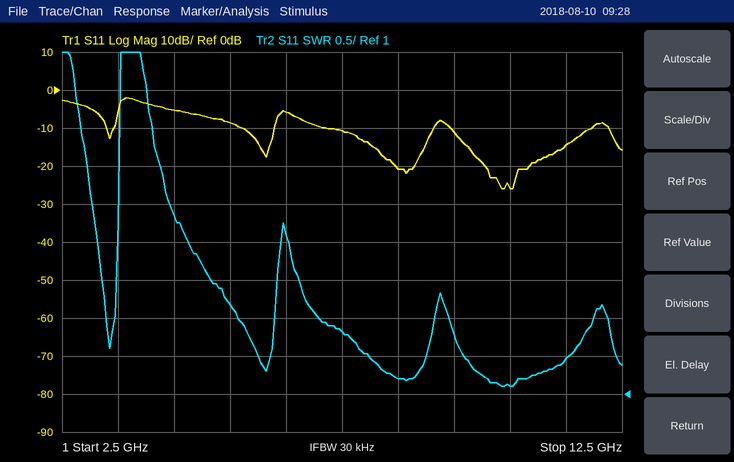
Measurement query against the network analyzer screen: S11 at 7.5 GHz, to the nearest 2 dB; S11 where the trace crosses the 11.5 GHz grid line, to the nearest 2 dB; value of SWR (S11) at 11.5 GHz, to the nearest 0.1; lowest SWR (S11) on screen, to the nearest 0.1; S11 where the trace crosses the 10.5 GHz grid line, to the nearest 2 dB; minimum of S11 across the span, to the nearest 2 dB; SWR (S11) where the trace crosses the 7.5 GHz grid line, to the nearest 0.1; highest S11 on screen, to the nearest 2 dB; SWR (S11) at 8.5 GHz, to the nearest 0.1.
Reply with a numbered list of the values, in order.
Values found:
1. -10 dB
2. -14 dB
3. 1.5
4. 1.1
5. -26 dB
6. -26 dB
7. 1.8
8. -2 dB
9. 1.2
